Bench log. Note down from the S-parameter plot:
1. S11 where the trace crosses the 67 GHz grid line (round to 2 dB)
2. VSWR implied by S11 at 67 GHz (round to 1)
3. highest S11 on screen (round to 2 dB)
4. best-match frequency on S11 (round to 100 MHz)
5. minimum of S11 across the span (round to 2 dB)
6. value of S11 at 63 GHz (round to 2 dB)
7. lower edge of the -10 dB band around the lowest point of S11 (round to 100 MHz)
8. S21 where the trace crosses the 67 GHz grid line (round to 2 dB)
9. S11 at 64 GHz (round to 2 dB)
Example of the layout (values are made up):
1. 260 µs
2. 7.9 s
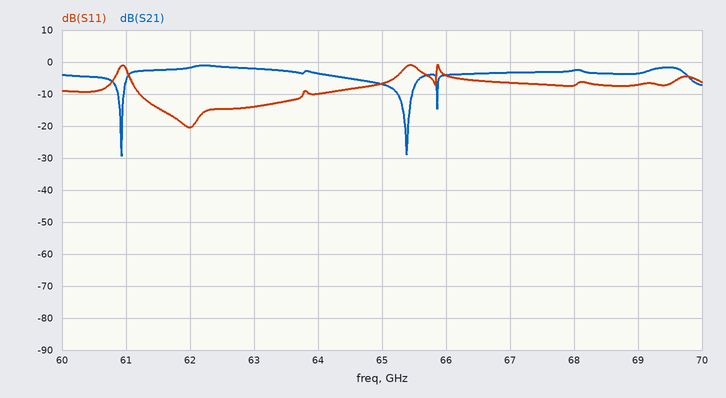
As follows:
1. -6 dB
2. 3
3. 0 dB
4. 62.0 GHz
5. -20 dB
6. -14 dB
7. 61.2 GHz
8. -4 dB
9. -10 dB
